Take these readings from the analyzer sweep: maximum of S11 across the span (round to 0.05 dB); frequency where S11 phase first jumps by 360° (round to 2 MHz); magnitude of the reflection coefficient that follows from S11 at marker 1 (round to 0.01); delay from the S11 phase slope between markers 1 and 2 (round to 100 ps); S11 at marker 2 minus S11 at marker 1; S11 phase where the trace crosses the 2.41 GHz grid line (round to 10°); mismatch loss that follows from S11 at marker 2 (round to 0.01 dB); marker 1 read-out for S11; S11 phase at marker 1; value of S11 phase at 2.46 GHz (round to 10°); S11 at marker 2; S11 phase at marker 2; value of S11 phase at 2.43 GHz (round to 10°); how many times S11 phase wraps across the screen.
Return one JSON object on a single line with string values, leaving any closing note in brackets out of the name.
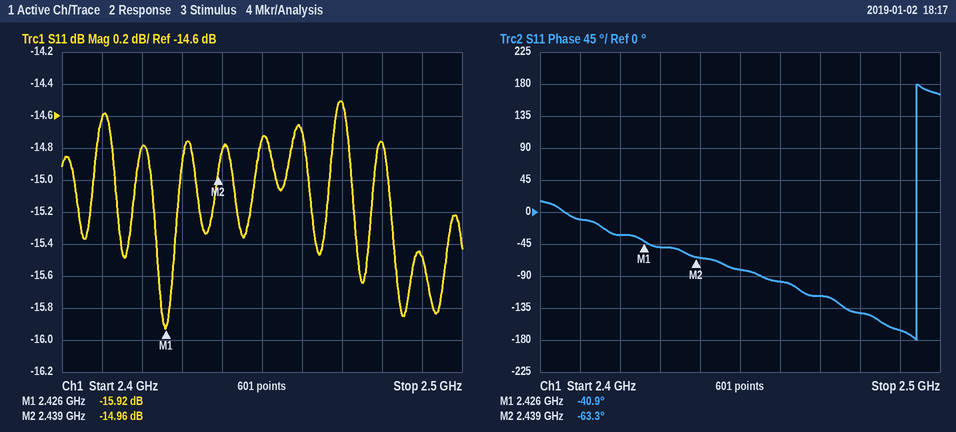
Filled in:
{"maximum of S11 across the span": "-14.50 dB", "frequency where S11 phase first jumps by 360°": "2.494 GHz", "magnitude of the reflection coefficient that follows from S11 at marker 1": "0.16", "delay from the S11 phase slope between markers 1 and 2": "4.8 ns", "S11 at marker 2 minus S11 at marker 1": "0.96 dB", "S11 phase where the trace crosses the 2.41 GHz grid line": "-10°", "mismatch loss that follows from S11 at marker 2": "0.14 dB", "marker 1 read-out for S11": "-15.92 dB", "S11 phase at marker 1": "-40.9°", "value of S11 phase at 2.46 GHz": "-100°", "S11 at marker 2": "-14.96 dB", "S11 phase at marker 2": "-63.3°", "value of S11 phase at 2.43 GHz": "-50°", "how many times S11 phase wraps across the screen": "1"}
